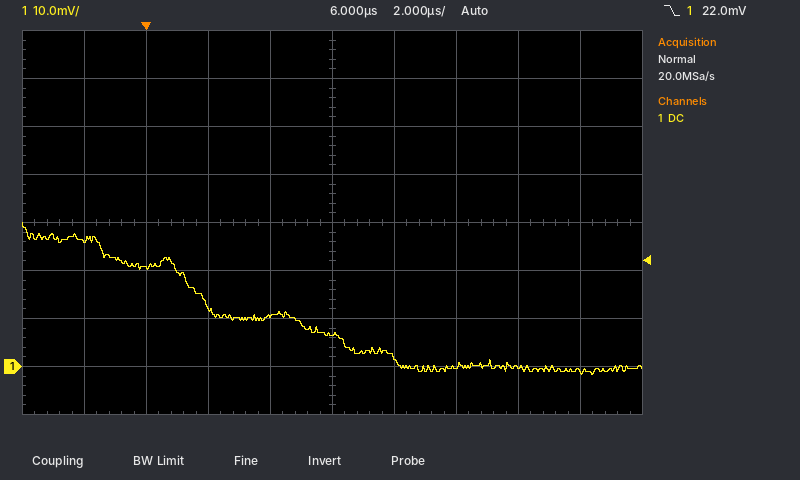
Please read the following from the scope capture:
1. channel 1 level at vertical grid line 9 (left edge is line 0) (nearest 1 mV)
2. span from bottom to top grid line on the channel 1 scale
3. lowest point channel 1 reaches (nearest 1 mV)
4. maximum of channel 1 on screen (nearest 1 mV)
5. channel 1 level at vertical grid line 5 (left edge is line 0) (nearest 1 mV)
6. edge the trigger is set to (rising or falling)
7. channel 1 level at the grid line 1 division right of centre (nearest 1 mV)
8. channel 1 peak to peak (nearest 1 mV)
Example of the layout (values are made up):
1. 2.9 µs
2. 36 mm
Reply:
1. -1 mV
2. 80 mV
3. -2 mV
4. 30 mV
5. 7 mV
6. falling
7. 2 mV
8. 32 mV
